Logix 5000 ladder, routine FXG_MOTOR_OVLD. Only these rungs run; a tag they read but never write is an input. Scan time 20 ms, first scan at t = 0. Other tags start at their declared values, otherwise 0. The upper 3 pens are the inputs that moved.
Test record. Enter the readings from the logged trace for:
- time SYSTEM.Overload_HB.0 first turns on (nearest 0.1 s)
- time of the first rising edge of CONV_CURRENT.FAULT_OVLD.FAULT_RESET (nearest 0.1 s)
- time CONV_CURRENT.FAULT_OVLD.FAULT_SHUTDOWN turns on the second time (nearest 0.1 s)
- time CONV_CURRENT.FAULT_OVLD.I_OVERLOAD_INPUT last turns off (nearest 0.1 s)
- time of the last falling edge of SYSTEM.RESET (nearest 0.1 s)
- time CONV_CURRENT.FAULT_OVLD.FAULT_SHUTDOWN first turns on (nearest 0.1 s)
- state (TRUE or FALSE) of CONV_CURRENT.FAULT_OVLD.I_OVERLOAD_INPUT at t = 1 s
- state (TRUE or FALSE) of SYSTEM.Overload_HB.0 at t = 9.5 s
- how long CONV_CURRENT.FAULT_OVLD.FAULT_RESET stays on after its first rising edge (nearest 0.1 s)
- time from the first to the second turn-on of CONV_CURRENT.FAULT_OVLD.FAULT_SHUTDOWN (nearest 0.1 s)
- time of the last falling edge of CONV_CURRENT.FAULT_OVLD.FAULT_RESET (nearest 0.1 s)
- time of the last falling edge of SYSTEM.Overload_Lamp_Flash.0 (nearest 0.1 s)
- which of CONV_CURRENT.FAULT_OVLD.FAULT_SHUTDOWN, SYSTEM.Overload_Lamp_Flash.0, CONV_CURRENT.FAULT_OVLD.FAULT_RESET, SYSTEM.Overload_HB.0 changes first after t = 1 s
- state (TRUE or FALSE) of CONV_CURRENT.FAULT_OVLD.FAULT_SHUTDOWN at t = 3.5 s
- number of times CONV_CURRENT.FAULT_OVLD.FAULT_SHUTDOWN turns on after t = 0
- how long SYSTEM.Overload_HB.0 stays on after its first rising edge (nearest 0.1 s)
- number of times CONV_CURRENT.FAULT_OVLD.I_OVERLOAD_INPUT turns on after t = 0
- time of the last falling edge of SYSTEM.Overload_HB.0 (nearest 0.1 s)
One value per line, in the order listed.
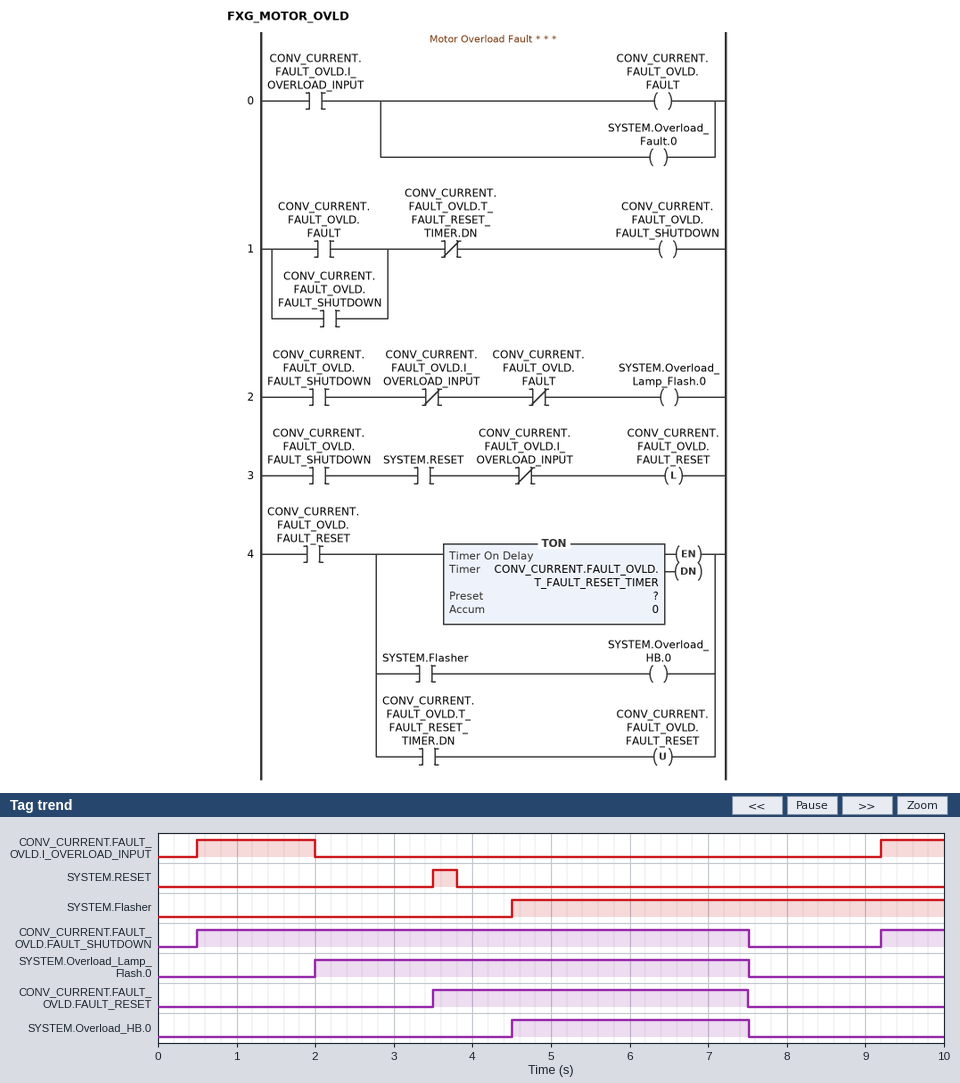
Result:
4.5 s
3.5 s
9.2 s
2.0 s
3.8 s
0.5 s
TRUE
FALSE
4.0 s
8.7 s
7.5 s
7.5 s
SYSTEM.Overload_Lamp_Flash.0
TRUE
2
3.0 s
2
7.5 s
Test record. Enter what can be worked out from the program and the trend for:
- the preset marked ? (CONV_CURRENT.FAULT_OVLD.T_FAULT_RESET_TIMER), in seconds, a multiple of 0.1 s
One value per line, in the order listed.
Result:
4.0 s
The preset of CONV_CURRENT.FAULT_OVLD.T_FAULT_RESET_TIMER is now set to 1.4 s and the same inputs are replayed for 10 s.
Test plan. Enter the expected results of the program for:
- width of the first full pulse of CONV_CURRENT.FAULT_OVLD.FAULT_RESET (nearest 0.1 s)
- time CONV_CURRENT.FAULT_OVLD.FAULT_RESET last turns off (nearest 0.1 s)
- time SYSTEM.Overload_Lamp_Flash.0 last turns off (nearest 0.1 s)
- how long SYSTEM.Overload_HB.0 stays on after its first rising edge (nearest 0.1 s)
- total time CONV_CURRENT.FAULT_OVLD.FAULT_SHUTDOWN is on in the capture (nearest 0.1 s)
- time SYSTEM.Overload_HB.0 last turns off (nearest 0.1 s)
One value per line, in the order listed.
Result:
1.4 s
4.9 s
4.9 s
0.4 s
5.2 s
4.9 s
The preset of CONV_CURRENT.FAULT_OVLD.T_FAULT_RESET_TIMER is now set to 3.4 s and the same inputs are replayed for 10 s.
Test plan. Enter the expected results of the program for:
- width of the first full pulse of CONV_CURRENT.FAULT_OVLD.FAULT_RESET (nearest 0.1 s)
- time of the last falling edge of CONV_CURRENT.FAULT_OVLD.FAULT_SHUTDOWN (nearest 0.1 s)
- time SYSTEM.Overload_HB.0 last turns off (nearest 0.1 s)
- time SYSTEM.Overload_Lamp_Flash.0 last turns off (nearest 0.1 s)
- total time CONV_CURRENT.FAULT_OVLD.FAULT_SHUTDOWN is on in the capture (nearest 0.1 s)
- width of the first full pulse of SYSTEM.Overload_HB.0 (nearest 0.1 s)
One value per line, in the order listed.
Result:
3.4 s
6.9 s
6.9 s
6.9 s
7.2 s
2.4 s
